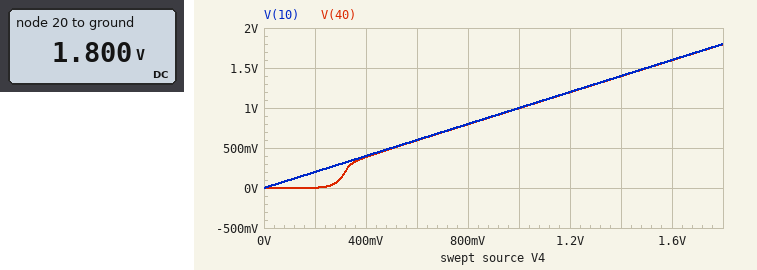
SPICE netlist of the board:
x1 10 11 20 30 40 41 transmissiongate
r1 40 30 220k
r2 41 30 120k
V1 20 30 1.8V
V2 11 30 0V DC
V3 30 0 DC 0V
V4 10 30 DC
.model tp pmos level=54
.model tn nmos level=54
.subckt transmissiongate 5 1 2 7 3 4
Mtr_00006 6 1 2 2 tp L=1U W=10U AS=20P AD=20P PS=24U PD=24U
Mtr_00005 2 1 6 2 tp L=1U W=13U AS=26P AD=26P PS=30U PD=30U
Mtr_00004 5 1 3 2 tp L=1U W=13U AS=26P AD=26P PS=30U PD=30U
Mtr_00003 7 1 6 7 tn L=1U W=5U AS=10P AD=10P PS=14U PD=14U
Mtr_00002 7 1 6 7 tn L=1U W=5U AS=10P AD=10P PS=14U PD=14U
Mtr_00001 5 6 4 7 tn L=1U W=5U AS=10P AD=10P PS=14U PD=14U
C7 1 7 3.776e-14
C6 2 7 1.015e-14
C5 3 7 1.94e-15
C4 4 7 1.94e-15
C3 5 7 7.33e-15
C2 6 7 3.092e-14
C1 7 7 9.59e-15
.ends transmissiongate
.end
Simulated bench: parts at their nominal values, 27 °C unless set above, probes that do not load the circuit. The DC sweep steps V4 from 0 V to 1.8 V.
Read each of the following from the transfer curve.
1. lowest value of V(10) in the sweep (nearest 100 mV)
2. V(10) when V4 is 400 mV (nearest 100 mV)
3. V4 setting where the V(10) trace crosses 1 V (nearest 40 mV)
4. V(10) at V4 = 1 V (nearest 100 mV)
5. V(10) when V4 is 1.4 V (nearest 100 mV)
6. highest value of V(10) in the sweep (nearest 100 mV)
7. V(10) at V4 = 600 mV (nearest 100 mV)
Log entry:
0 V
400 mV
1.00 V
1.0 V
1.4 V
1.8 V
600 mV
